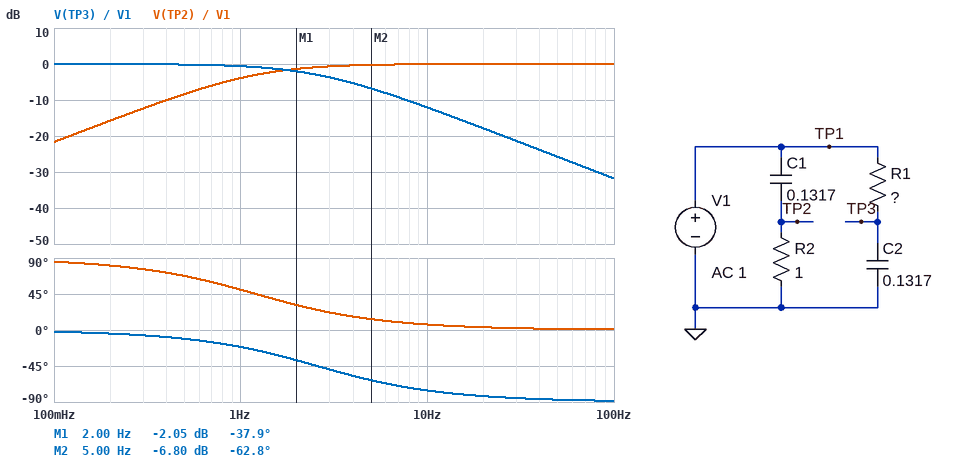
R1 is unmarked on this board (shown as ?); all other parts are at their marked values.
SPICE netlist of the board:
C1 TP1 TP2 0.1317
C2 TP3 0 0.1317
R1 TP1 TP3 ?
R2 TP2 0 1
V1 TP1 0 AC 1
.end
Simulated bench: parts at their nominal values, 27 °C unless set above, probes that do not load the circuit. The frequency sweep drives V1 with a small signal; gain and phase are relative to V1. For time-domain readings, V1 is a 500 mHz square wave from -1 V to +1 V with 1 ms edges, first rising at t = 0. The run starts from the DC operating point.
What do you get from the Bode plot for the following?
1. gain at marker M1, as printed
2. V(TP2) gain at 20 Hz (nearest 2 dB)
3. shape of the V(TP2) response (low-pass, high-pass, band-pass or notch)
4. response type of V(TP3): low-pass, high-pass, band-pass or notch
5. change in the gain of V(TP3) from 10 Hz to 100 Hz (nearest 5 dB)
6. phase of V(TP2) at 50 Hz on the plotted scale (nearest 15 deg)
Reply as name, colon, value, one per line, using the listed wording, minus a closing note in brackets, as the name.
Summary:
gain at marker M1, as printed: -2.05 dB
V(TP2) gain at 20 Hz: 0 dB
shape of the V(TP2) response: high-pass
response type of V(TP3): low-pass, high-pass, band-pass or notch: low-pass
change in the gain of V(TP3) from 10 Hz to 100 Hz: -20 dB
phase of V(TP2) at 50 Hz on the plotted scale: 0 deg
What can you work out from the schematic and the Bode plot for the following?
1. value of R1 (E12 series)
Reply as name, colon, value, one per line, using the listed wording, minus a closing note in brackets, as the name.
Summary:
value of R1: 0.47 Ω
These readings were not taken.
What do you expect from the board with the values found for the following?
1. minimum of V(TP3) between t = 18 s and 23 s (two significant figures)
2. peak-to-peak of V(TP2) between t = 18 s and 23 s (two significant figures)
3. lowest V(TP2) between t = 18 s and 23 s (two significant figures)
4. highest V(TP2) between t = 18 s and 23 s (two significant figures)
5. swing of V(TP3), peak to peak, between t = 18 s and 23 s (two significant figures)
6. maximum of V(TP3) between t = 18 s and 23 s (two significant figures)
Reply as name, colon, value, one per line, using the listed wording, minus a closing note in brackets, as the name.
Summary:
minimum of V(TP3) between t = 18 s and 23 s: -1.0 V
peak-to-peak of V(TP2) between t = 18 s and 23 s: 4.0 V
lowest V(TP2) between t = 18 s and 23 s: -2.0 V
highest V(TP2) between t = 18 s and 23 s: 2.0 V
swing of V(TP3), peak to peak, between t = 18 s and 23 s: 2.0 V
maximum of V(TP3) between t = 18 s and 23 s: 1.0 V
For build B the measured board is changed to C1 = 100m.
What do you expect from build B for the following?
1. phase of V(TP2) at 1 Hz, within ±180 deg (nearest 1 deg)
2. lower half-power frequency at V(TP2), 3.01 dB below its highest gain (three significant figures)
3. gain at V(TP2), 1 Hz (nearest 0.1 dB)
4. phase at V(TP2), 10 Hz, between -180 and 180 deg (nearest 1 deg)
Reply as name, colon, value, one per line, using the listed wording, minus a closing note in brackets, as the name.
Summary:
phase of V(TP2) at 1 Hz, within ±180 deg: 58 deg
lower half-power frequency at V(TP2), 3.01 dB below its highest gain: 1.59 Hz
gain at V(TP2), 1 Hz: -5.5 dB
phase at V(TP2), 10 Hz, between -180 and 180 deg: 9 deg
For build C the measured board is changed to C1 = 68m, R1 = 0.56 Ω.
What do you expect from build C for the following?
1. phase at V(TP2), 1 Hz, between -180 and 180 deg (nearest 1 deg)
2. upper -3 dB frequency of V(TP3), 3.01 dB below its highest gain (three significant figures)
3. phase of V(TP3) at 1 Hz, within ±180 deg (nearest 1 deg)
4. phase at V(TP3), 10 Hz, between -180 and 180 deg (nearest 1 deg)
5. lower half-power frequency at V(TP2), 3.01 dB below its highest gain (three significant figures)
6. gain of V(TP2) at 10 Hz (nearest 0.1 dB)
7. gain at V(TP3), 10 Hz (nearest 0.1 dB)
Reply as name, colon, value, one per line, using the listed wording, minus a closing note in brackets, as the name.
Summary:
phase at V(TP2), 1 Hz, between -180 and 180 deg: 67 deg
upper -3 dB frequency of V(TP3), 3.01 dB below its highest gain: 2.16 Hz
phase of V(TP3) at 1 Hz, within ±180 deg: -25 deg
phase at V(TP3), 10 Hz, between -180 and 180 deg: -78 deg
lower half-power frequency at V(TP2), 3.01 dB below its highest gain: 2.34 Hz
gain of V(TP2) at 10 Hz: -0.2 dB
gain at V(TP3), 10 Hz: -13.5 dB
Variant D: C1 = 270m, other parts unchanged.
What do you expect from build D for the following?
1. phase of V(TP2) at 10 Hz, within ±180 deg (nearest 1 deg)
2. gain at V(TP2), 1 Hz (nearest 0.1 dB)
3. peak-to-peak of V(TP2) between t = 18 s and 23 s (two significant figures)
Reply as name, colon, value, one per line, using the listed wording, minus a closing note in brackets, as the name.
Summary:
phase of V(TP2) at 10 Hz, within ±180 deg: 3 deg
gain at V(TP2), 1 Hz: -1.3 dB
peak-to-peak of V(TP2) between t = 18 s and 23 s: 3.9 V
